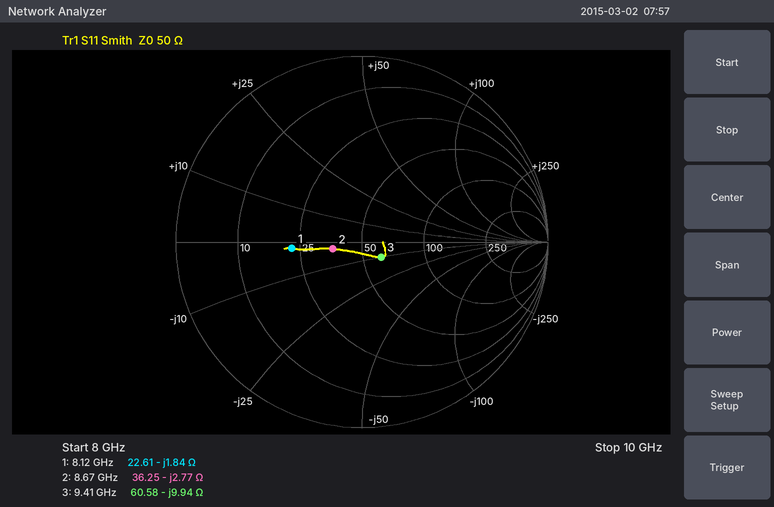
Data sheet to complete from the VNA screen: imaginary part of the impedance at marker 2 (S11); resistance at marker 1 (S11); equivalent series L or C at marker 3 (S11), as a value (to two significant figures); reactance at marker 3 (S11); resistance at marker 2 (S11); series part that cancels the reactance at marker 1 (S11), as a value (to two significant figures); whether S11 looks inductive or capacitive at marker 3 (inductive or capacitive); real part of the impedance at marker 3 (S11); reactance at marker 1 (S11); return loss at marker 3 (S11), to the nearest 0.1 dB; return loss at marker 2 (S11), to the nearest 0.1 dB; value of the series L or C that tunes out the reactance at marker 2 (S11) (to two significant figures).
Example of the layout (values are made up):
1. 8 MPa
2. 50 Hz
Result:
1. -2.77 Ω
2. 22.61 Ω
3. 1.7 pF
4. -9.94 Ω
5. 36.25 Ω
6. 36 pH
7. capacitive
8. 60.58 Ω
9. -1.84 Ω
10. 17.7 dB
11. 15.8 dB
12. 51 pH
